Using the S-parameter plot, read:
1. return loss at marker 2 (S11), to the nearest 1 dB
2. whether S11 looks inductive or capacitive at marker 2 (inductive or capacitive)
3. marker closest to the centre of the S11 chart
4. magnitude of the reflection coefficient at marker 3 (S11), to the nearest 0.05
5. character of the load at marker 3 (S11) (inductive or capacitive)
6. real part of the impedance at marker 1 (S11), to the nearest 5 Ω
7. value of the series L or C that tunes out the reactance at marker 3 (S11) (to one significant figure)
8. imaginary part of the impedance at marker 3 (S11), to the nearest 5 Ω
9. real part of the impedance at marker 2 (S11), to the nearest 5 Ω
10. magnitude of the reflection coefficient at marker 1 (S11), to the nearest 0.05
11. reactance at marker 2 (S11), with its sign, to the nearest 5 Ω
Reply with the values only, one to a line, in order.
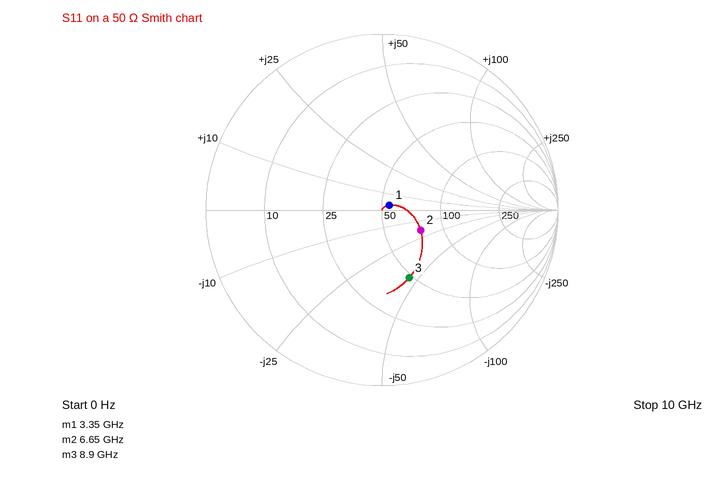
12 dB
capacitive
marker 1
0.40
capacitive
55 Ω
800 pH
-45 Ω
75 Ω
0.05
-20 Ω
